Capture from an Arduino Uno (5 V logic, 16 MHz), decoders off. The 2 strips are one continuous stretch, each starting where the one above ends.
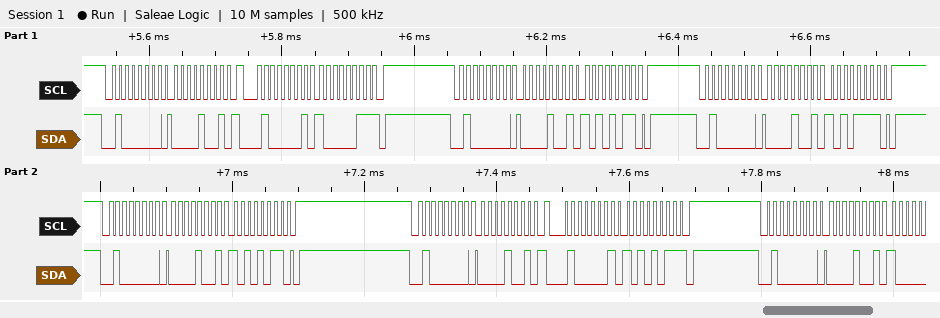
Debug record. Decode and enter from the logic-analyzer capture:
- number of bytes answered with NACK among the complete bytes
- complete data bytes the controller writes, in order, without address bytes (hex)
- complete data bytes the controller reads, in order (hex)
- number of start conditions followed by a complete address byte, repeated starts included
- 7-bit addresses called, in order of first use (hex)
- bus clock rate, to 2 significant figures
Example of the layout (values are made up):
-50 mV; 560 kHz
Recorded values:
2; 09 09 AB 09 AF 09 AB 09 09; 83 AB; 8; 0x20; 100 kHz
